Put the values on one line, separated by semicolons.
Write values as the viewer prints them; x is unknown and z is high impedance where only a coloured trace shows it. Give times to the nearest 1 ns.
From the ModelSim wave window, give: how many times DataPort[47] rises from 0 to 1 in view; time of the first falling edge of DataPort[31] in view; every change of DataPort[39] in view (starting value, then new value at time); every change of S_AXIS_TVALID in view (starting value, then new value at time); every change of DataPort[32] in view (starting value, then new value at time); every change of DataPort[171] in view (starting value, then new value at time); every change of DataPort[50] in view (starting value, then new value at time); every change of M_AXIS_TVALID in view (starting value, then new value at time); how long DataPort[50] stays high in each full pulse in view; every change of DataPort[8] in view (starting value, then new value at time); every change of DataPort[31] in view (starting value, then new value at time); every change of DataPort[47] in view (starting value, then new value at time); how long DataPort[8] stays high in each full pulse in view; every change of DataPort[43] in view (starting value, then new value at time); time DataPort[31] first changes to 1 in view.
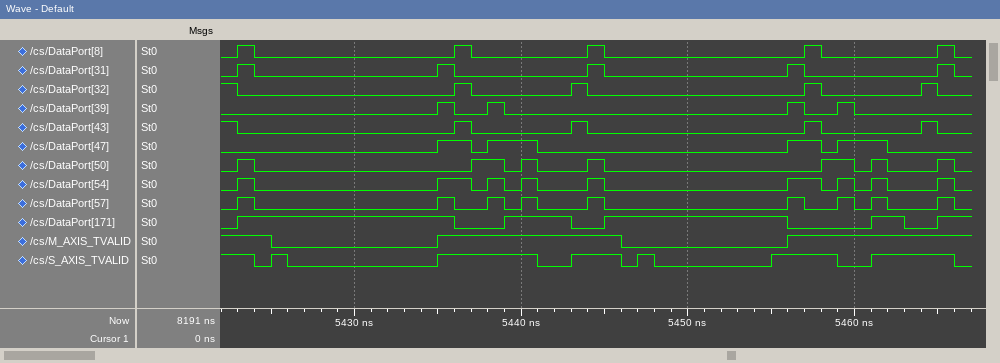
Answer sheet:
4; 5424 ns; 0, 1 at 5435 ns, 0 at 5436 ns, 1 at 5438 ns, 0 at 5439 ns, 1 at 5456 ns, 0 at 5457 ns, 1 at 5459 ns, 0 at 5460 ns; 1, 0 at 5424 ns, 1 at 5425 ns, 0 at 5426 ns, 1 at 5435 ns, 0 at 5441 ns, 1 at 5443 ns, 0 at 5446 ns, 1 at 5447 ns, 0 at 5448 ns, 1 at 5455 ns, 0 at 5459 ns, 1 at 5461 ns, 0 at 5466 ns; 1, 0 at 5423 ns, 1 at 5436 ns, 0 at 5437 ns, 1 at 5443 ns, 0 at 5444 ns, 1 at 5457 ns, 0 at 5458 ns, 1 at 5464 ns, 0 at 5465 ns; 0, 1 at 5423 ns, 0 at 5436 ns, 1 at 5439 ns, 0 at 5443 ns, 1 at 5445 ns, 0 at 5456 ns, 1 at 5461 ns, 0 at 5463 ns, 1 at 5465 ns; 0, 1 at 5423 ns, 0 at 5424 ns, 1 at 5437 ns, 0 at 5439 ns, 1 at 5440 ns, 0 at 5441 ns, 1 at 5444 ns, 0 at 5445 ns, 1 at 5458 ns, 0 at 5460 ns, 1 at 5461 ns, 0 at 5462 ns, 1 at 5465 ns, 0 at 5466 ns; 1, 0 at 5425 ns, 1 at 5435 ns, 0 at 5446 ns, 1 at 5456 ns; 1 ns, 2 ns, 1 ns, 1 ns, 2 ns, 1 ns, 1 ns; 0, 1 at 5423 ns, 0 at 5424 ns, 1 at 5436 ns, 0 at 5437 ns, 1 at 5444 ns, 0 at 5445 ns, 1 at 5457 ns, 0 at 5458 ns, 1 at 5465 ns, 0 at 5466 ns; 0, 1 at 5423 ns, 0 at 5424 ns, 1 at 5435 ns, 0 at 5436 ns, 1 at 5444 ns, 0 at 5445 ns, 1 at 5456 ns, 0 at 5457 ns, 1 at 5465 ns, 0 at 5466 ns; 0, 1 at 5435 ns, 0 at 5437 ns, 1 at 5438 ns, 0 at 5441 ns, 1 at 5456 ns, 0 at 5458 ns, 1 at 5459 ns, 0 at 5462 ns; 1 ns, 1 ns, 1 ns, 1 ns, 1 ns; 1, 0 at 5423 ns, 1 at 5436 ns, 0 at 5437 ns, 1 at 5443 ns, 0 at 5444 ns, 1 at 5457 ns, 0 at 5458 ns, 1 at 5464 ns, 0 at 5465 ns; 5423 ns
